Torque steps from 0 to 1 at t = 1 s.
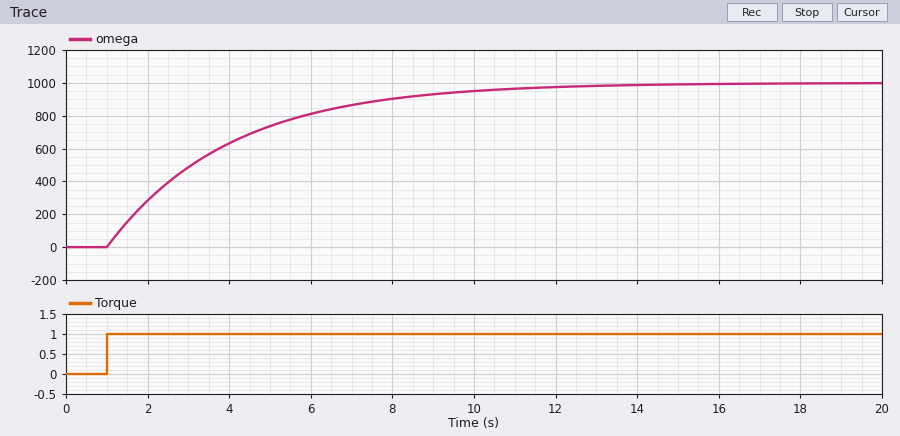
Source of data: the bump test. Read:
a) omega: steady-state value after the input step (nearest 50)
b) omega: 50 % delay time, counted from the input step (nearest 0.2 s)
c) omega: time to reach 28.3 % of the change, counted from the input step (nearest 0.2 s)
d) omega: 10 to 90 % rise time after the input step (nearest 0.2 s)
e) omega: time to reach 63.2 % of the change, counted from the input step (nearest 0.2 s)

1000
2.0 s
1.0 s
6.6 s
3.0 s
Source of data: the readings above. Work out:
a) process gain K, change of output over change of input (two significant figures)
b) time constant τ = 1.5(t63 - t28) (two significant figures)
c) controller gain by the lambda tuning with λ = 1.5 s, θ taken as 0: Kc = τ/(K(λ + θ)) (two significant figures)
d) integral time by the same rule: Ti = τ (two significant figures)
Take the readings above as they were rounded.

1000
3.0 s
0.0020
3.0 s
